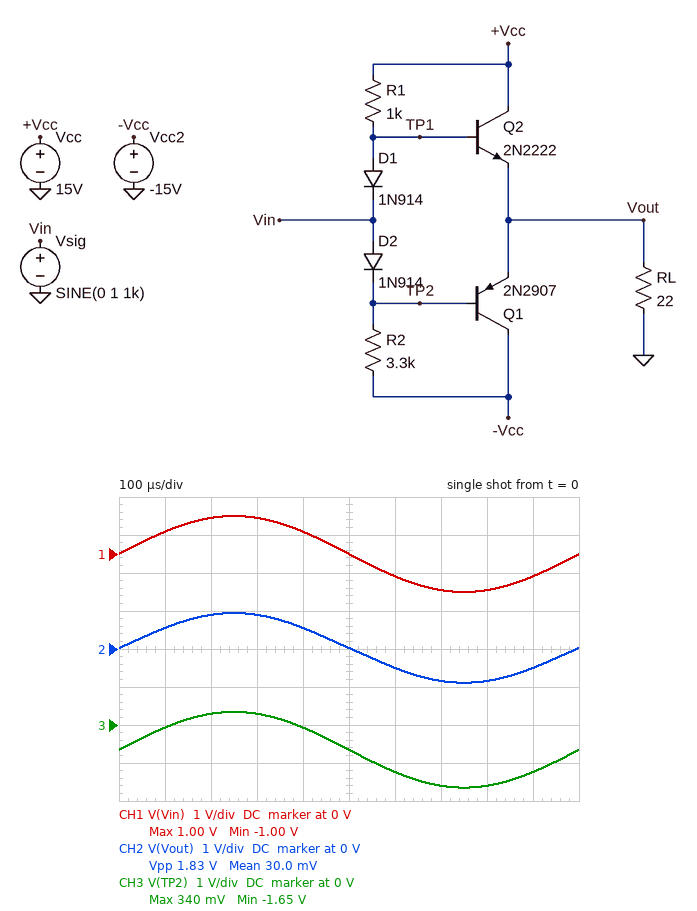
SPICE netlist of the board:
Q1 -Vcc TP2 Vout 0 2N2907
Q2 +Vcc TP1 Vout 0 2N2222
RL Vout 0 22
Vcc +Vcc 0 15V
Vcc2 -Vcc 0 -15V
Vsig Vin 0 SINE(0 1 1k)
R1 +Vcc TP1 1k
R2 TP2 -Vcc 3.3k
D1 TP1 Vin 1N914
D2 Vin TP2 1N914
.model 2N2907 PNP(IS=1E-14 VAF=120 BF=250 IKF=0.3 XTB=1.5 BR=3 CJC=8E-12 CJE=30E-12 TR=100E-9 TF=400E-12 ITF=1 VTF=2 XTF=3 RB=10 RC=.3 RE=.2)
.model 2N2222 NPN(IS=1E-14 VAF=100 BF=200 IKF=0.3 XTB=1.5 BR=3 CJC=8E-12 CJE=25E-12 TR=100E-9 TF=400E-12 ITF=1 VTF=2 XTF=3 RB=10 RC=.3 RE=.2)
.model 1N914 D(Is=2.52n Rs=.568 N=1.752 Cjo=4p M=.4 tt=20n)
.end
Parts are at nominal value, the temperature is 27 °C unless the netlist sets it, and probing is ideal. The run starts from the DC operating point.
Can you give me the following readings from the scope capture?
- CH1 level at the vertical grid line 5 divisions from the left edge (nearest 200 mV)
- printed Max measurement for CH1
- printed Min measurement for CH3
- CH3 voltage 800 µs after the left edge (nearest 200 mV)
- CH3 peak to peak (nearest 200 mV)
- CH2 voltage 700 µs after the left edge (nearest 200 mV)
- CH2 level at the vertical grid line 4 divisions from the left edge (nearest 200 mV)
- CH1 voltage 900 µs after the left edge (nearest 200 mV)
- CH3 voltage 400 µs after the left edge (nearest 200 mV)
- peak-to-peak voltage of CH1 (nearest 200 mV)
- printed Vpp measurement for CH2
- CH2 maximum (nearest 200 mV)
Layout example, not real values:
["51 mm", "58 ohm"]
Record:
["0 V", "1.00 V", "-1.65 V", "-1.6 V", "2.0 V", "-800 mV", "600 mV", "-600 mV", "0 V", "2.0 V", "1.83 V", "1.0 V"]
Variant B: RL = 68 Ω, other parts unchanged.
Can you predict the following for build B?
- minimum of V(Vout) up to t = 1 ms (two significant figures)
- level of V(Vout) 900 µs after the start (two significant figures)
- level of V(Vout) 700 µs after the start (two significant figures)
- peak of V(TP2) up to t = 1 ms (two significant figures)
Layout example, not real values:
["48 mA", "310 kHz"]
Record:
["-920 mV", "-530 mV", "-880 mV", "340 mV"]
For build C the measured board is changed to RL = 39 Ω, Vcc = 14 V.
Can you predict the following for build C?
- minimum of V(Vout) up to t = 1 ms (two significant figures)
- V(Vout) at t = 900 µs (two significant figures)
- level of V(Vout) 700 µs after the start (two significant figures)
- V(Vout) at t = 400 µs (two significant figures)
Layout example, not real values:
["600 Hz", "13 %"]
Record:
["-910 mV", "-510 mV", "-860 mV", "570 mV"]
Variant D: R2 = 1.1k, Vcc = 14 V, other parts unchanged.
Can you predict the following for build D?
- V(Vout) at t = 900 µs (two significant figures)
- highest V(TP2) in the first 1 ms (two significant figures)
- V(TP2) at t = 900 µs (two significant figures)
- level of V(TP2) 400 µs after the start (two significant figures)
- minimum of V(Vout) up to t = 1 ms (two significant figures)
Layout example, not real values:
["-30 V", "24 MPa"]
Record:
["-550 mV", "290 mV", "-1.3 V", "-120 mV", "-940 mV"]
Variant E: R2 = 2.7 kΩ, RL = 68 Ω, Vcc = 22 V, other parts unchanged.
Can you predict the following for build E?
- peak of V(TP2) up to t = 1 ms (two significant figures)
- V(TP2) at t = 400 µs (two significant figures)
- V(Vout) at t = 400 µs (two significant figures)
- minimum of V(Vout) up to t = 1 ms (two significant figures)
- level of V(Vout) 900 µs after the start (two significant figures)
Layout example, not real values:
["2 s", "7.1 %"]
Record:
["330 mV", "-77 mV", "600 mV", "-930 mV", "-530 mV"]
